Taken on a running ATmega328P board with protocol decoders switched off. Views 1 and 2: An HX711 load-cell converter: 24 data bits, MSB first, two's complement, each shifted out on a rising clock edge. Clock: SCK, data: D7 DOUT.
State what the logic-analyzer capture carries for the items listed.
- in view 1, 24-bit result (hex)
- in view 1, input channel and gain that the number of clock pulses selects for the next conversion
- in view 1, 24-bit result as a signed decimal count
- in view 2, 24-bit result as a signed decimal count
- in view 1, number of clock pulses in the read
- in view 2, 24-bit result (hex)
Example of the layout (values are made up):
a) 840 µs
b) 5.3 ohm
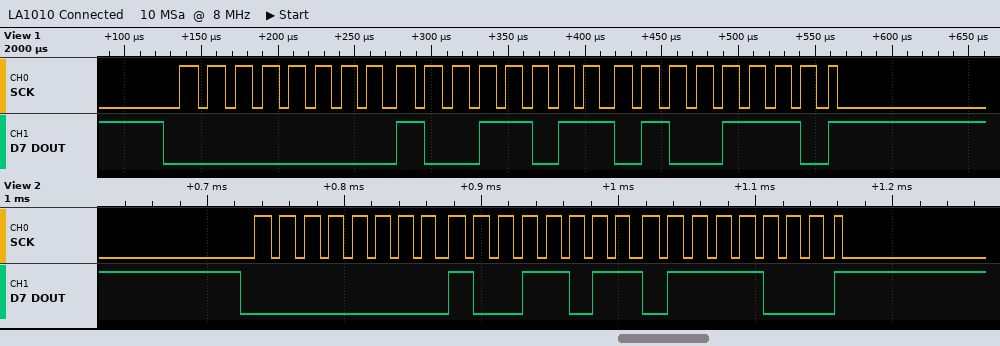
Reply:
a) 0x009B4E
b) channel A, gain 128
c) 39758
d) 39800
e) 25
f) 0x009B78
